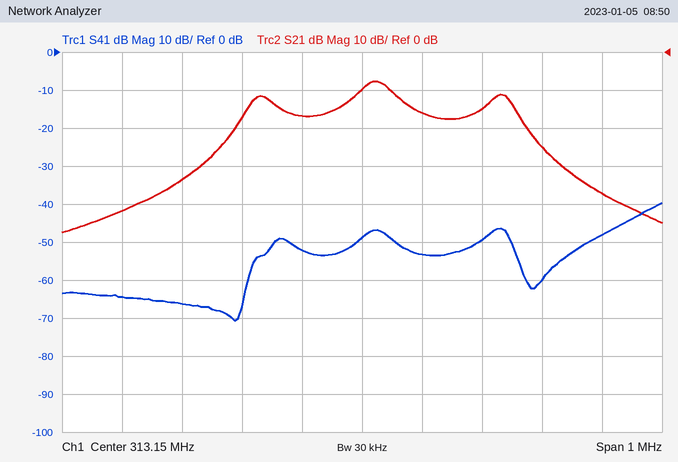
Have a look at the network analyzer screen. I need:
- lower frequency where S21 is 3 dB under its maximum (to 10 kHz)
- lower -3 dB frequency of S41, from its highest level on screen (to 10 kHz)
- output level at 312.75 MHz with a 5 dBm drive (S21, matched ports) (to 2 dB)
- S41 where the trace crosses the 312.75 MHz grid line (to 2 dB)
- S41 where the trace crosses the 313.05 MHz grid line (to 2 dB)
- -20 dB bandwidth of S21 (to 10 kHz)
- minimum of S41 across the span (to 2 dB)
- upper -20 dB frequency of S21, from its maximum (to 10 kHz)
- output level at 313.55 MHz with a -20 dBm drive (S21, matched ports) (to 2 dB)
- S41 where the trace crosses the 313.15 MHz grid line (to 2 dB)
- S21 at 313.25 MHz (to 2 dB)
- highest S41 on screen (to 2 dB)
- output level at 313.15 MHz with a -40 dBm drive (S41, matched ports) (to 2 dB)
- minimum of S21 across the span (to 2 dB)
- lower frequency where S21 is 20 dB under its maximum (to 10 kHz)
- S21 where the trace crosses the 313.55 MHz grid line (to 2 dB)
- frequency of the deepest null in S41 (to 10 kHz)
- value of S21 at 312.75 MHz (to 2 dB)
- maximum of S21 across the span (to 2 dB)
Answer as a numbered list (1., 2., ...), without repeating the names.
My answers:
1. 313.14 MHz
2. 313.61 MHz
3. -36 dBm
4. -64 dB
5. -52 dB
6. 570 kHz
7. -70 dB
8. 313.47 MHz
9. -58 dBm
10. -48 dB
11. -16 dB
12. -40 dB
13. -88 dBm
14. -48 dB
15. 312.90 MHz
16. -38 dB
17. 312.94 MHz
18. -42 dB
19. -8 dB
